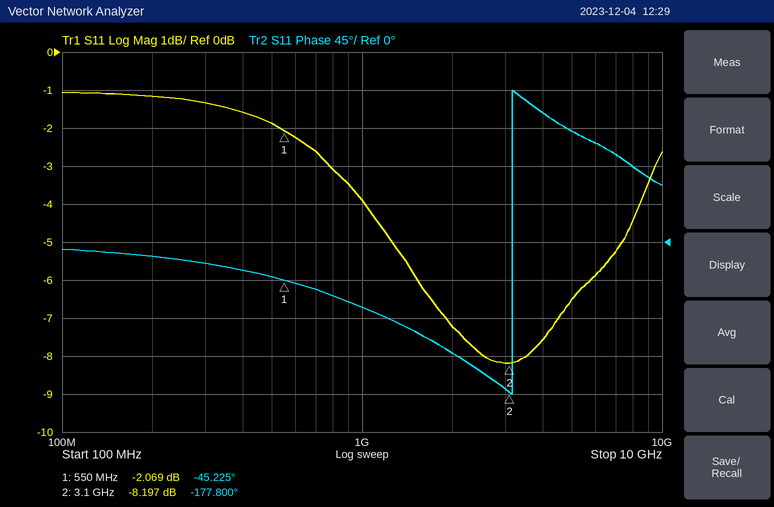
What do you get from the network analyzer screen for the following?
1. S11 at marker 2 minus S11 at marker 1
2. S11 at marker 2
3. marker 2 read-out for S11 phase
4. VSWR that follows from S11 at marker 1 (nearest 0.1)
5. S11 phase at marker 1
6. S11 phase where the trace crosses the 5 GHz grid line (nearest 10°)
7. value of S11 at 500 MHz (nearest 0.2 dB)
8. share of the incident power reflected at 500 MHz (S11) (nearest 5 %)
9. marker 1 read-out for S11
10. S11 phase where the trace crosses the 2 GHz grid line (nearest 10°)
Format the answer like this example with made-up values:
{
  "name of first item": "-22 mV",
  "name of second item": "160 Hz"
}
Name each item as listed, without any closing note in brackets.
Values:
{
  "S11 at marker 2 minus S11 at marker 1": "-6.128 dB",
  "S11 at marker 2": "-8.197 dB",
  "marker 2 read-out for S11 phase": "-177.800°",
  "VSWR that follows from S11 at marker 1": "8.4",
  "S11 phase at marker 1": "-45.225°",
  "S11 phase where the trace crosses the 5 GHz grid line": "130°",
  "value of S11 at 500 MHz": "-1.8 dB",
  "share of the incident power reflected at 500 MHz (S11)": "65 %",
  "marker 1 read-out for S11": "-2.069 dB",
  "S11 phase where the trace crosses the 2 GHz grid line": "-130°"
}
